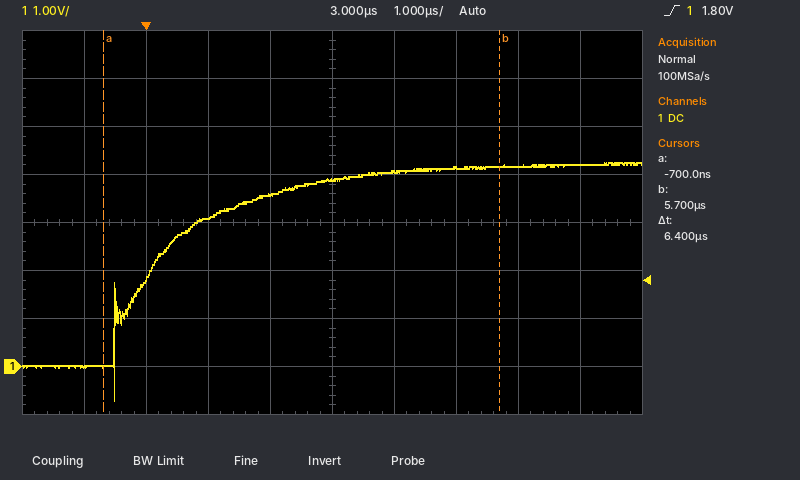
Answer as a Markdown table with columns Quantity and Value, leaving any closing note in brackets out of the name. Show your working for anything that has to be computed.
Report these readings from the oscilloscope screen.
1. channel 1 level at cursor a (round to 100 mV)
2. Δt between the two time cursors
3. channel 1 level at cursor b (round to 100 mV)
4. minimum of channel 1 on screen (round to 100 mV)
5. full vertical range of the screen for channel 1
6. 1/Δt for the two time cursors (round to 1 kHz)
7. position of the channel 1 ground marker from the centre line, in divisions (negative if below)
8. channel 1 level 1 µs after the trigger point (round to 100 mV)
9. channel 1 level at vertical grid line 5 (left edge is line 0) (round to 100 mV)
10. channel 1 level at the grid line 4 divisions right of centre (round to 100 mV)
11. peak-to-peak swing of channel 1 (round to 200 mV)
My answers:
| Quantity | Value |
|---|---|
| channel 1 level at cursor a | 0.0 V |
| Δt between the two time cursors | 6.4 µs |
| channel 1 level at cursor b | 4.2 V |
| minimum of channel 1 on screen | -700 mV |
| full vertical range of the screen for channel 1 | 8 V |
| 1/Δt for the two time cursors | 1 / 6.4 µs ≈ 156 kHz |
| position of the channel 1 ground marker from the centre line, in divisions | -3.0 div |
| channel 1 level 1 µs after the trigger point | 3.1 V |
| channel 1 level at vertical grid line 5 (left edge is line 0) | 3.9 V |
| channel 1 level at the grid line 4 divisions right of centre | 4.2 V |
| peak-to-peak swing of channel 1 | 5.0 V |
